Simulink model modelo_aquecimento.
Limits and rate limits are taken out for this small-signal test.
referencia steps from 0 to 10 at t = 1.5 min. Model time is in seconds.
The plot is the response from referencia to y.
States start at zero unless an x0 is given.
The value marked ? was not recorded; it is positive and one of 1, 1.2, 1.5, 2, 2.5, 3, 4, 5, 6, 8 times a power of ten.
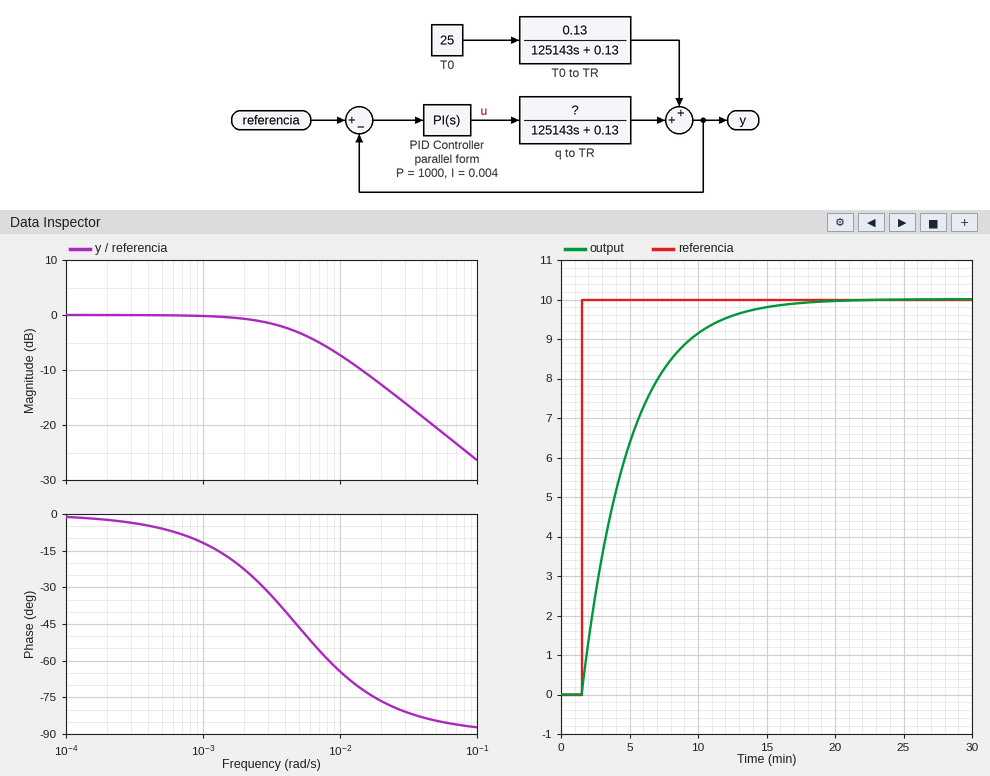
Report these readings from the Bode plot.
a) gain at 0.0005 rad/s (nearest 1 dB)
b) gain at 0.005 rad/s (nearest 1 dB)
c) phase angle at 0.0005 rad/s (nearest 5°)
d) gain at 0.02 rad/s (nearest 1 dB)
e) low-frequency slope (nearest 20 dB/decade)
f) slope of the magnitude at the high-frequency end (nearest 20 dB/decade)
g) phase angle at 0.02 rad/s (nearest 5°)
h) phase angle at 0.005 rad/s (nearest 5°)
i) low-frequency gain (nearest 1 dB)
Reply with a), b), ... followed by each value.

a) 0 dB
b) -3 dB
c) -5°
d) -13 dB
e) 0 dB/decade
f) -20 dB/decade
g) -75°
h) -45°
i) 0 dB
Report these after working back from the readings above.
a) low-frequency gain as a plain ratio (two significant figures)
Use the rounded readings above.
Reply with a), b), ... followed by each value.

a) 1.0
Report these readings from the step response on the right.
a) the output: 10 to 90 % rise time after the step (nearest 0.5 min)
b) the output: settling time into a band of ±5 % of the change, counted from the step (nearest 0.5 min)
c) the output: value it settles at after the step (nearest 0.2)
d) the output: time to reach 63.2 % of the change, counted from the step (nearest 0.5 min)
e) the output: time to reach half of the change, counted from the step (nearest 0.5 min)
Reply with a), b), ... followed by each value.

a) 7.5 min
b) 10.5 min
c) 10.0
d) 3.5 min
e) 2.5 min
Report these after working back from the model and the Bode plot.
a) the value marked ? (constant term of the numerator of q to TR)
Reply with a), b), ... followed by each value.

a) 0.6
